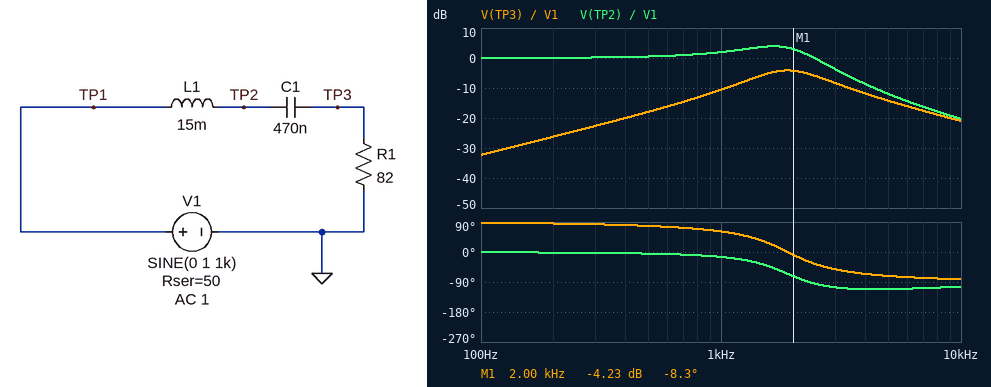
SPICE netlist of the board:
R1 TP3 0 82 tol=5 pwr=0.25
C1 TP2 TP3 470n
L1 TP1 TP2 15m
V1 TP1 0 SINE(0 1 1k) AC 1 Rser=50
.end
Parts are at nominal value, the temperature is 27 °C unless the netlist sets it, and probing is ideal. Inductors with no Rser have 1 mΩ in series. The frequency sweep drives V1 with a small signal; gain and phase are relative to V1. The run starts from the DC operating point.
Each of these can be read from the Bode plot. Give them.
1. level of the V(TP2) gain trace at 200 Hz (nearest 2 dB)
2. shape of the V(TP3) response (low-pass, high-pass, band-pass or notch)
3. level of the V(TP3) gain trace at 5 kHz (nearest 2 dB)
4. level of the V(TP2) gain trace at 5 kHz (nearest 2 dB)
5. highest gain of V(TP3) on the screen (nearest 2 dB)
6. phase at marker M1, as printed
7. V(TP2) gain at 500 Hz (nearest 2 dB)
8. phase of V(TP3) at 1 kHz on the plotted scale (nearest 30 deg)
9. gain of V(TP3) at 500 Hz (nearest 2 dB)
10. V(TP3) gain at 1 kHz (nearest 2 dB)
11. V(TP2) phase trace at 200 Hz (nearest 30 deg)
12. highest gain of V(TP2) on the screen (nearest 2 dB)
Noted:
0 dB
band-pass
-14 dB
-12 dB
-4 dB
-8.3 deg
0 dB
60 deg
-18 dB
-10 dB
0 deg
4 dB
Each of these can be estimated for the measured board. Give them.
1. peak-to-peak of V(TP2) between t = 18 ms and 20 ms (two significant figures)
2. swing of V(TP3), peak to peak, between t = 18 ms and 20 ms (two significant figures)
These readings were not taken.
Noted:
2.5 V
590 mV
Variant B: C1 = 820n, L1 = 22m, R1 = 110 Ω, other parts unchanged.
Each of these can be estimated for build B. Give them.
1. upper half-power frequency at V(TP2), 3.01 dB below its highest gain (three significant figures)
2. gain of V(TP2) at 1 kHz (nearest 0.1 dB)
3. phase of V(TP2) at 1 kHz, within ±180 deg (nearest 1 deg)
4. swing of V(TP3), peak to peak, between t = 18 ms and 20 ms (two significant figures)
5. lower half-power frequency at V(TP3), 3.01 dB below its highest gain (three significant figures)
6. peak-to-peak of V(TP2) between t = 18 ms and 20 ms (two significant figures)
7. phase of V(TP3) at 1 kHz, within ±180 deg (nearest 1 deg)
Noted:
1.52 kHz
2.4 dB
-41 deg
1.3 V
740 Hz
2.6 V
19 deg
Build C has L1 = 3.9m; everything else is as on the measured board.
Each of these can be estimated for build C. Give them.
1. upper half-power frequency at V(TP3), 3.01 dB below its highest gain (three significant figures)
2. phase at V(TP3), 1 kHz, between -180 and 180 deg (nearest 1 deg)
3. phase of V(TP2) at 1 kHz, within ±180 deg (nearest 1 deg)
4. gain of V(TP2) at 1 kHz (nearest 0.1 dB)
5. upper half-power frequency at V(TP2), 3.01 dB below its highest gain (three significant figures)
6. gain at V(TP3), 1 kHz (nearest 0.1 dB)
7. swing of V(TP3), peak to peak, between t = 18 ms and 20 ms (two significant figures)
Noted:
7.28 kHz
67 deg
-9 deg
0.2 dB
4.99 kHz
-12.4 dB
480 mV
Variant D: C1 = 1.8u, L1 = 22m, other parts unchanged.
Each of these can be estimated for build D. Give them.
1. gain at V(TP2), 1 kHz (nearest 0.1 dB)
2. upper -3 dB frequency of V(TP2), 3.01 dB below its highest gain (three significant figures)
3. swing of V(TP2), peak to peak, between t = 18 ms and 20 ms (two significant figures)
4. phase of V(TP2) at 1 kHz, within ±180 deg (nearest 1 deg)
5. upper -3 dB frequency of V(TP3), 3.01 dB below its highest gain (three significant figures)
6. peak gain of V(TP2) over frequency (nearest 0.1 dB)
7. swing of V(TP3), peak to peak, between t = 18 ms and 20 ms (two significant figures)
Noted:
-1.4 dB
1.04 kHz
1.7 V
-68 deg
1.41 kHz
1.2 dB
1.2 V
